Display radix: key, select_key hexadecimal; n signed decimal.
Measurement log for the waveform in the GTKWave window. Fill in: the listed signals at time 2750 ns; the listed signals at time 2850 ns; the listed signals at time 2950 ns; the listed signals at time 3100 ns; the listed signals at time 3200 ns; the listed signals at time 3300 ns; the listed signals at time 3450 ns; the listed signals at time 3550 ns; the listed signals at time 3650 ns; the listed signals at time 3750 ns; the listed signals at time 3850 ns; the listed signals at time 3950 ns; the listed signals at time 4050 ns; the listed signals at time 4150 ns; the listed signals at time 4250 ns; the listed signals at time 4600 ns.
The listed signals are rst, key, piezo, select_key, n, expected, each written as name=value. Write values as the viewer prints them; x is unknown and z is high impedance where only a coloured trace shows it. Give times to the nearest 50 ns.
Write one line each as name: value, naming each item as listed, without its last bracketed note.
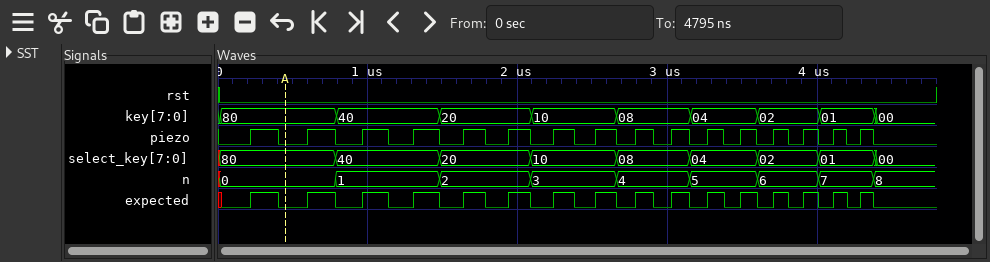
the listed signals at time 2750 ns: rst=0, key=08, piezo=0, select_key=08, n=4, expected=0
the listed signals at time 2850 ns: rst=0, key=08, piezo=1, select_key=08, n=4, expected=1
the listed signals at time 2950 ns: rst=0, key=08, piezo=0, select_key=08, n=4, expected=0
the listed signals at time 3100 ns: rst=0, key=08, piezo=1, select_key=08, n=4, expected=1
the listed signals at time 3200 ns: rst=0, key=04, piezo=0, select_key=04, n=5, expected=0
the listed signals at time 3300 ns: rst=0, key=04, piezo=1, select_key=04, n=5, expected=1
the listed signals at time 3450 ns: rst=0, key=04, piezo=0, select_key=04, n=5, expected=0
the listed signals at time 3550 ns: rst=0, key=04, piezo=1, select_key=04, n=5, expected=1
the listed signals at time 3650 ns: rst=0, key=02, piezo=0, select_key=02, n=6, expected=0
the listed signals at time 3750 ns: rst=0, key=02, piezo=1, select_key=02, n=6, expected=1
the listed signals at time 3850 ns: rst=0, key=02, piezo=0, select_key=02, n=6, expected=0
the listed signals at time 3950 ns: rst=0, key=02, piezo=1, select_key=02, n=6, expected=1
the listed signals at time 4050 ns: rst=0, key=01, piezo=0, select_key=01, n=7, expected=0
the listed signals at time 4150 ns: rst=0, key=01, piezo=1, select_key=01, n=7, expected=1
the listed signals at time 4250 ns: rst=0, key=01, piezo=0, select_key=01, n=7, expected=0
the listed signals at time 4600 ns: rst=0, key=00, piezo=0, select_key=00, n=8, expected=0
